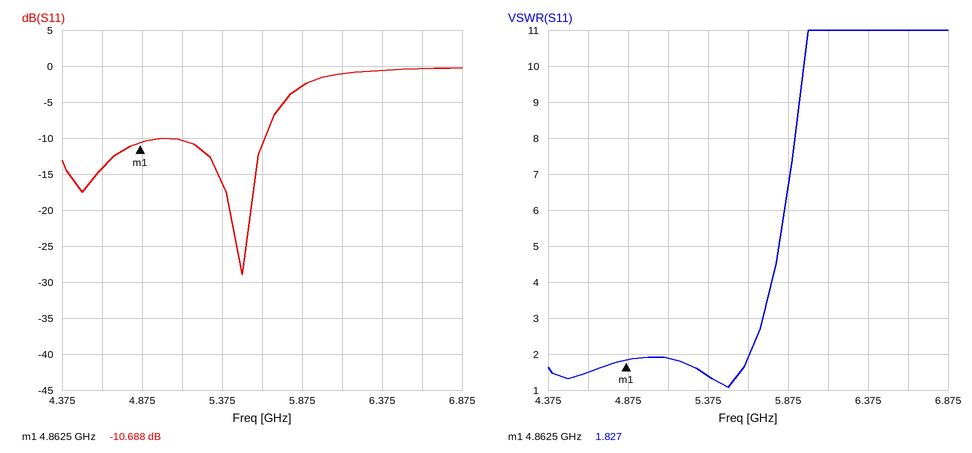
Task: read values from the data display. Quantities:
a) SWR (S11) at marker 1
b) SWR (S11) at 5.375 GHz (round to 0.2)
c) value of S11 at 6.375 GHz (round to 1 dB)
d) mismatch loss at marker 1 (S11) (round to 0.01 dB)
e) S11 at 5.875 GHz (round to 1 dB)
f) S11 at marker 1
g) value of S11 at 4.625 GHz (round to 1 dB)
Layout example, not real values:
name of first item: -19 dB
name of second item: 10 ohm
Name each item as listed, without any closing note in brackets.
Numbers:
SWR (S11) at marker 1: 1.827
SWR (S11) at 5.375 GHz: 1.4
value of S11 at 6.375 GHz: -1 dB
mismatch loss at marker 1 (S11): 0.39 dB
S11 at 5.875 GHz: -3 dB
S11 at marker 1: -10.688 dB
value of S11 at 4.625 GHz: -14 dB
